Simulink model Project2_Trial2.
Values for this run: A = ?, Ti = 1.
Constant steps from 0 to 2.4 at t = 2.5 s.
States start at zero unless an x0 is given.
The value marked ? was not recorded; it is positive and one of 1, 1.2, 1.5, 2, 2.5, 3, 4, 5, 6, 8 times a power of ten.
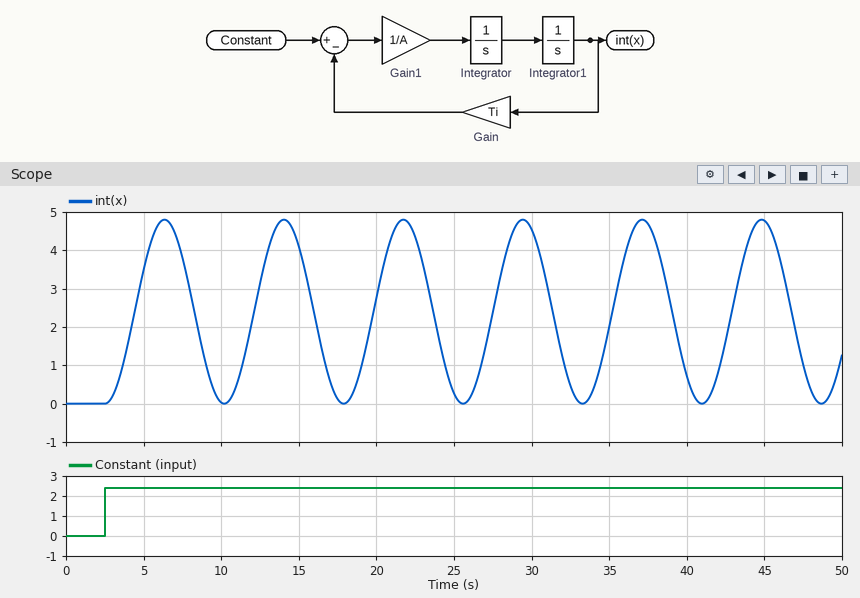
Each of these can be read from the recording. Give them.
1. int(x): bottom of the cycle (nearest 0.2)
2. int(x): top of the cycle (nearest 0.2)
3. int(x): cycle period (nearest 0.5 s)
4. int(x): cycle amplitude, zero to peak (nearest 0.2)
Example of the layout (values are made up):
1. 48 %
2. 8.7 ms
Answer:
1. 0.0
2. 4.8
3. 7.5 s
4. 2.4
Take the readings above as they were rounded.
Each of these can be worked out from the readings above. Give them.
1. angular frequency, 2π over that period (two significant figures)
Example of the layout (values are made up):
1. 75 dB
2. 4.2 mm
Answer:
1. 0.84 rad/s
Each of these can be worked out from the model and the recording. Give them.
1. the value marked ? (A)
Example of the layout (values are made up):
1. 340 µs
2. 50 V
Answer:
1. 1.5
